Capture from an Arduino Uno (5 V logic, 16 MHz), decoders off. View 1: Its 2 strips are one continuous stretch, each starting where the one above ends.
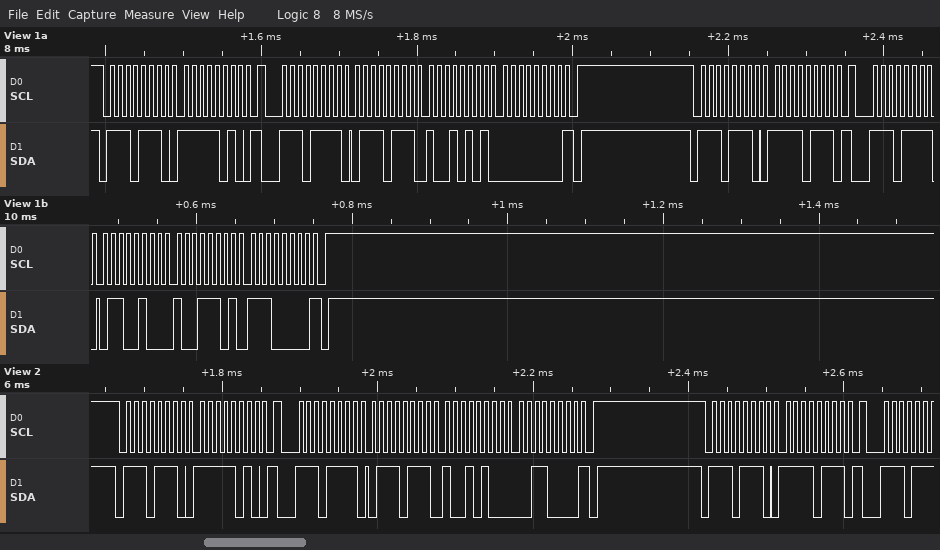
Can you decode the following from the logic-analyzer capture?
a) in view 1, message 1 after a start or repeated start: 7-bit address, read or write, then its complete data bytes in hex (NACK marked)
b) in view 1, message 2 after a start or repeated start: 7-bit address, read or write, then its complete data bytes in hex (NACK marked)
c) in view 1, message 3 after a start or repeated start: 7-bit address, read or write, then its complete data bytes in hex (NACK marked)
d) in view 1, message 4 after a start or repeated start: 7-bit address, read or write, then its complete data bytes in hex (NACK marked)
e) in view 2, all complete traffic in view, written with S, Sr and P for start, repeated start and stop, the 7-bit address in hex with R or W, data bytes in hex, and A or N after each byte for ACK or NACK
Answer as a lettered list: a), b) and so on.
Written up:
a) 0x77 write: FA
b) 0x77 read: 77 95 00 NACK
c) 0x77 write: F7
d) 0x77 read: 64 9D E0 NACK
e) S 77W A FA A Sr 77R A 77 A 94 A 30 N P S 77W A F7 A
